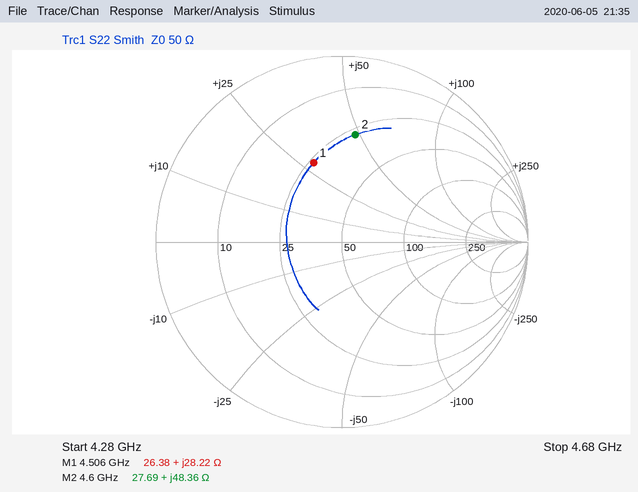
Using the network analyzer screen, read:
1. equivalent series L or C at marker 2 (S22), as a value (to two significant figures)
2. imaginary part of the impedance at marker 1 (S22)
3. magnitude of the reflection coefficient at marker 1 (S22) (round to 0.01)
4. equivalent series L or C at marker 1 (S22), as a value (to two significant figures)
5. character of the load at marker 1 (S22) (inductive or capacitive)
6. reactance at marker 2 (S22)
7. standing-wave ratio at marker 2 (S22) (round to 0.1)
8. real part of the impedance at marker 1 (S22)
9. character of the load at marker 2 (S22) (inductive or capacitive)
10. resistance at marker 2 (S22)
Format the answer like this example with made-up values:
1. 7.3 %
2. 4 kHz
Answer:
1. 1.7 nH
2. +28.22 Ω
3. 0.45
4. 1.00 nH
5. inductive
6. +48.36 Ω
7. 3.8
8. 26.38 Ω
9. inductive
10. 27.69 Ω
